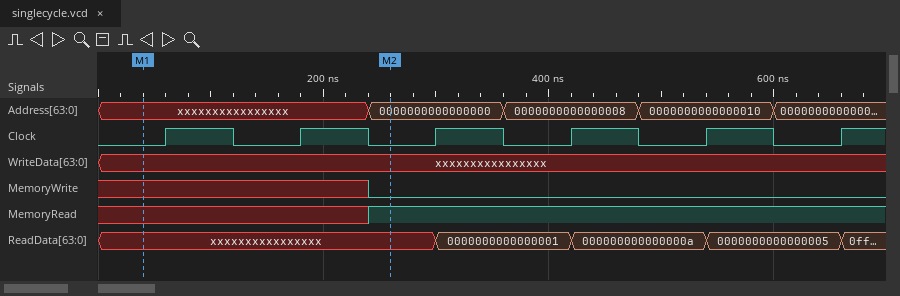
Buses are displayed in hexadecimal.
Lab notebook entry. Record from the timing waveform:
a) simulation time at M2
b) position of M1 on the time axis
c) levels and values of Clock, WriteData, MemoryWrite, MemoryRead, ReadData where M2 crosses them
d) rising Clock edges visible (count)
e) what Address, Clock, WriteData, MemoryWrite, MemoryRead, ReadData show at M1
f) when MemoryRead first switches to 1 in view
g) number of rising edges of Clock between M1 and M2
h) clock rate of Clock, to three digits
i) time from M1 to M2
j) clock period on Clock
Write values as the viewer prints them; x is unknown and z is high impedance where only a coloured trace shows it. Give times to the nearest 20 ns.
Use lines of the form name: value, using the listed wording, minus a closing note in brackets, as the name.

simulation time at M2: 260 ns
position of M1 on the time axis: 40 ns
levels and values of Clock, WriteData, MemoryWrite, MemoryRead, ReadData where M2 crosses them: Clock=0, WriteData=xxxxxxxxxxxxxxxx, MemoryWrite=0, MemoryRead=1, ReadData=xxxxxxxxxxxxxxxx
rising Clock edges visible: 6
what Address, Clock, WriteData, MemoryWrite, MemoryRead, ReadData show at M1: Address=xxxxxxxxxxxxxxxx, Clock=0, WriteData=xxxxxxxxxxxxxxxx, MemoryWrite=x, MemoryRead=x, ReadData=xxxxxxxxxxxxxxxx
when MemoryRead first switches to 1 in view: 240 ns
number of rising edges of Clock between M1 and M2: 2
clock rate of Clock, to three digits: 8.33 MHz
time from M1 to M2: 220 ns
clock period on Clock: 120 ns
